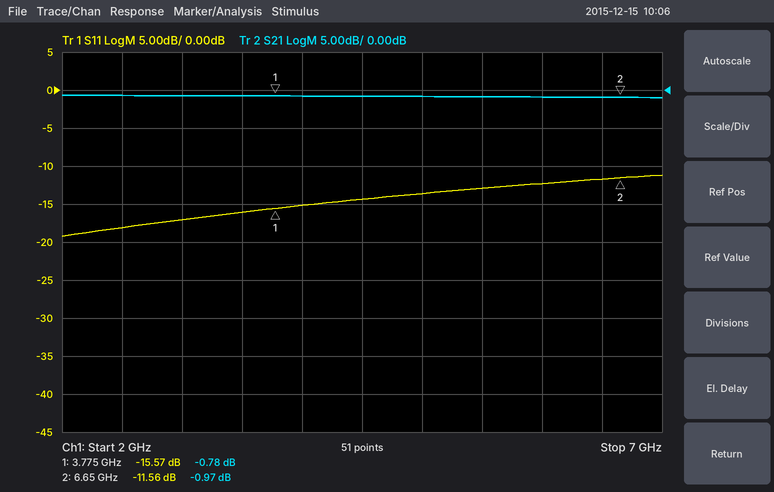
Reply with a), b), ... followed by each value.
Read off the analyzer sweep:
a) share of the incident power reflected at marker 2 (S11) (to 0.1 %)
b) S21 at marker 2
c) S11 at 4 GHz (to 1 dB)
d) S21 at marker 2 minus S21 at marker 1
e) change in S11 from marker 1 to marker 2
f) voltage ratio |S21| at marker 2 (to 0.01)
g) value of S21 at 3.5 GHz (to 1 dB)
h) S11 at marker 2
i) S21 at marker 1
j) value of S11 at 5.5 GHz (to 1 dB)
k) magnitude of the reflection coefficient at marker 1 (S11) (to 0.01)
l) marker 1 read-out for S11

a) 7.0 %
b) -0.97 dB
c) -15 dB
d) -0.19 dB
e) 4.01 dB
f) 0.89
g) -1 dB
h) -11.56 dB
i) -0.78 dB
j) -13 dB
k) 0.17
l) -15.57 dB
